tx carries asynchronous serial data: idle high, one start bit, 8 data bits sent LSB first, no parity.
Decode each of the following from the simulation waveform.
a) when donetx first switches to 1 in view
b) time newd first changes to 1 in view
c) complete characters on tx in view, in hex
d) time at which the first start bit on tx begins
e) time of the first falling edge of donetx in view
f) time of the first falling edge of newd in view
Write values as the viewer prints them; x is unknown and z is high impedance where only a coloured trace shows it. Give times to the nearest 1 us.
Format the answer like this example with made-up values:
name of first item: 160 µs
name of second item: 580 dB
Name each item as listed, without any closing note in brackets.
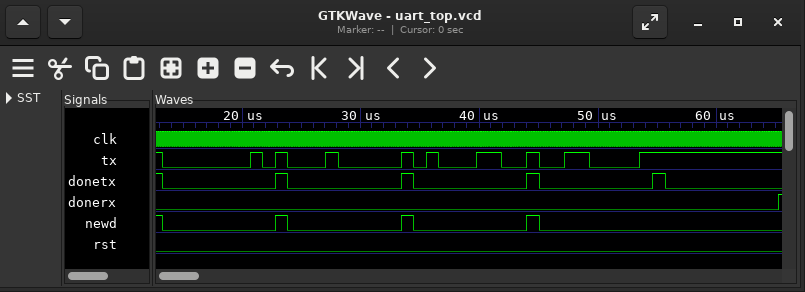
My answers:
when donetx first switches to 1 in view: 23 us
time newd first changes to 1 in view: 23 us
complete characters on tx in view, in hex: 40, 04, 31, 86
time at which the first start bit on tx begins: 13 us
time of the first falling edge of donetx in view: 13 us
time of the first falling edge of newd in view: 13 us
